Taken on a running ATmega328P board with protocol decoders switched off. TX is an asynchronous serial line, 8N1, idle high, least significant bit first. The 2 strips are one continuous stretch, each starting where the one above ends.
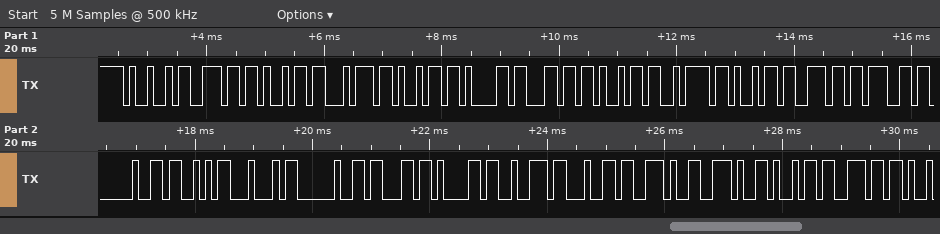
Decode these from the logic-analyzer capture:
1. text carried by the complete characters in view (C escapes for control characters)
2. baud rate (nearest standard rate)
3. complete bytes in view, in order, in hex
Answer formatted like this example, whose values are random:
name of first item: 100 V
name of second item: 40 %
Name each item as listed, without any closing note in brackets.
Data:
text carried by the complete characters in view: "Initializing SD card..in"
baud rate: 9600 baud
complete bytes in view, in order, in hex: 49 6E 69 74 69 61 6C 69 7A 69 6E 67 20 53 44 20 63 61 72 64 2E 2E 69 6E
